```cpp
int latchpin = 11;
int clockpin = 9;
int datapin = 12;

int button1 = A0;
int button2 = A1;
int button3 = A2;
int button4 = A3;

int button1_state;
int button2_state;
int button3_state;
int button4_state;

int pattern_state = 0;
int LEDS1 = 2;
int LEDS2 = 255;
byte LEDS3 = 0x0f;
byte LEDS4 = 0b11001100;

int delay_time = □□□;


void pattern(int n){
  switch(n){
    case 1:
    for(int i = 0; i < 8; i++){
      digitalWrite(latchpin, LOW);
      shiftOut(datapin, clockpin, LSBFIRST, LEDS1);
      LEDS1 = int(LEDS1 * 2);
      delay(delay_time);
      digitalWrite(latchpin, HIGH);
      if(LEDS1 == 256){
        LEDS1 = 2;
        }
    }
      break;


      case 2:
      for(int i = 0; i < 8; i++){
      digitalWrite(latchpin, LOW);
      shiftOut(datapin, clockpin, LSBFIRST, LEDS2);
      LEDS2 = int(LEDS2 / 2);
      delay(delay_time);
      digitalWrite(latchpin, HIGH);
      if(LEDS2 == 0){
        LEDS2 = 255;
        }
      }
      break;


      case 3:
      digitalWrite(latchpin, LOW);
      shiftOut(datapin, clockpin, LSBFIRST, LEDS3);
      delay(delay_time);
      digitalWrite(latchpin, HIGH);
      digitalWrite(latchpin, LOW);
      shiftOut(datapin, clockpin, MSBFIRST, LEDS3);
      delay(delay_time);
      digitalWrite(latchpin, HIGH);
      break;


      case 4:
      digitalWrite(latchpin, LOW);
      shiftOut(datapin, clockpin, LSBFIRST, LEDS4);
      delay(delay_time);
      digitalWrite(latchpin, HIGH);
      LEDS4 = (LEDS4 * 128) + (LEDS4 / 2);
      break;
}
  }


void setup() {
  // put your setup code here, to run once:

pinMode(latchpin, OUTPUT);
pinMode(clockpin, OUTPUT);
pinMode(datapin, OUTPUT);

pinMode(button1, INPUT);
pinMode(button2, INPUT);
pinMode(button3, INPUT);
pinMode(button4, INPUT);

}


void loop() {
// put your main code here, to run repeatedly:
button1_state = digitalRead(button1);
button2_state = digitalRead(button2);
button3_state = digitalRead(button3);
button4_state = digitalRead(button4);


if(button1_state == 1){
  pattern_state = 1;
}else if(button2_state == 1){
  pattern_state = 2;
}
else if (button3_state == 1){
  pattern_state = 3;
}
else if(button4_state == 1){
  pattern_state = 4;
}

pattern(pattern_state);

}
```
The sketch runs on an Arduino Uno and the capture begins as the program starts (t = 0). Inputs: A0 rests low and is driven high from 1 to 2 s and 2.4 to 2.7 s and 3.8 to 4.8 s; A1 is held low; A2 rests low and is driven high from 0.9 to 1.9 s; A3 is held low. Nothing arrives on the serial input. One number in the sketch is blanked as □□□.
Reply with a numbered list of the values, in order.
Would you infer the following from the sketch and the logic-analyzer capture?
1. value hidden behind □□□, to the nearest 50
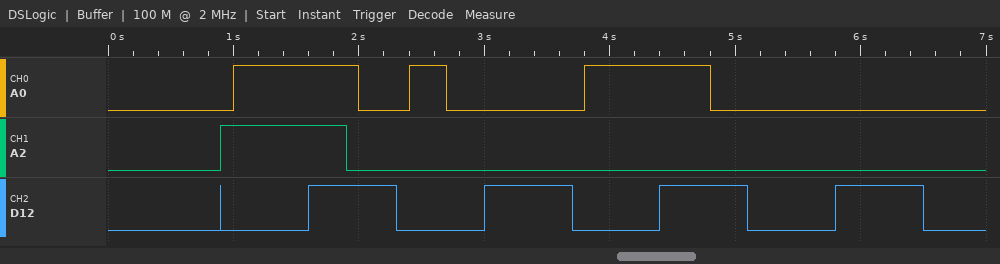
1. 700
